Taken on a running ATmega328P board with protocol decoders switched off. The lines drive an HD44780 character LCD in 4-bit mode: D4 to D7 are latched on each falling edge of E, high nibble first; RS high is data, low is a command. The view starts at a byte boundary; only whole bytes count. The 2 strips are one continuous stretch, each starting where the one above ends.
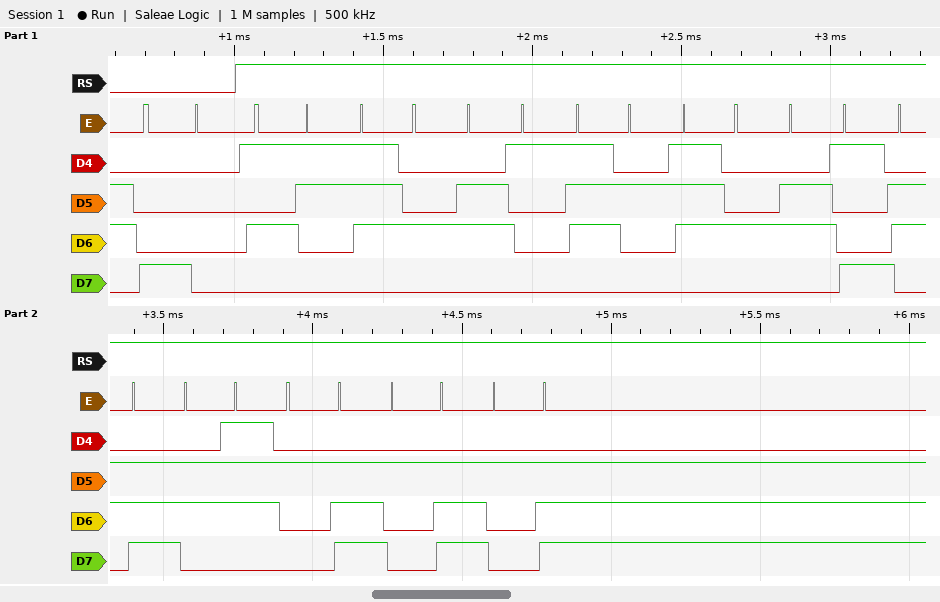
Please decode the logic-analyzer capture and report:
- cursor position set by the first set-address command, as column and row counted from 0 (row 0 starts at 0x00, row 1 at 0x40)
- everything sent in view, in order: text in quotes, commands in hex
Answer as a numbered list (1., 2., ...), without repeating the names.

1. column 0, row 0
2. 0x80 "Starting..."
